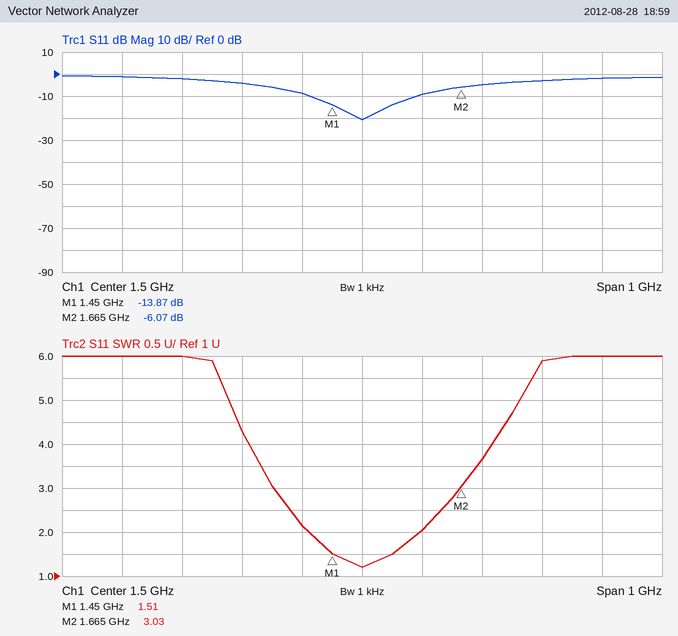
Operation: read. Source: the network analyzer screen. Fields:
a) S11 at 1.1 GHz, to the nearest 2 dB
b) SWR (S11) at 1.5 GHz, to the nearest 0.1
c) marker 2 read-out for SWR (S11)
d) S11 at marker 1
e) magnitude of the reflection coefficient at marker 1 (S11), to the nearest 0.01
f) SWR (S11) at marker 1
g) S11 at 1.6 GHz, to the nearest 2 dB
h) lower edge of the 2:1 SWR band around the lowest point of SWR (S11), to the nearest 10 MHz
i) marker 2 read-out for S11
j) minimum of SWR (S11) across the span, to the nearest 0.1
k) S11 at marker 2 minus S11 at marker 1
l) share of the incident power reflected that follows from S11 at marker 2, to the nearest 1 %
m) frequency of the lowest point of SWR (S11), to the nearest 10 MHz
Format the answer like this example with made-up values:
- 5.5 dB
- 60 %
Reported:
- -2 dB
- 1.2
- 3.03
- -13.87 dB
- 0.20
- 1.51
- -10 dB
- 1.41 GHz
- -6.07 dB
- 1.2
- 7.80 dB
- 25 %
- 1.50 GHz
